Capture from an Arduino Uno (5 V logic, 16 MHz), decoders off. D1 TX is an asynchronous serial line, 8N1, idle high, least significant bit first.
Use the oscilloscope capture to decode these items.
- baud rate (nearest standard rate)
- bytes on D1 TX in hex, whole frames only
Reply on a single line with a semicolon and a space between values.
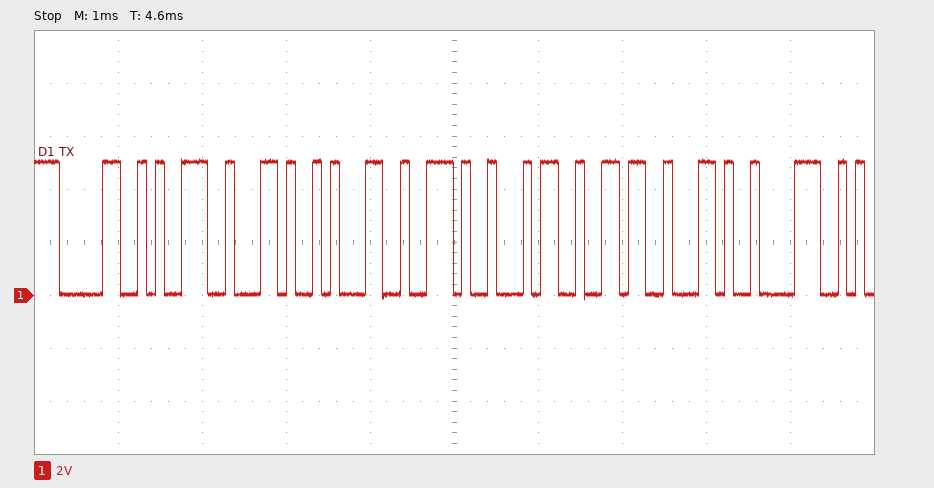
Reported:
9600 baud; 0x30 0x39 0x2C 0x31 0x2E 0x34 0x36 0x2C 0x38
